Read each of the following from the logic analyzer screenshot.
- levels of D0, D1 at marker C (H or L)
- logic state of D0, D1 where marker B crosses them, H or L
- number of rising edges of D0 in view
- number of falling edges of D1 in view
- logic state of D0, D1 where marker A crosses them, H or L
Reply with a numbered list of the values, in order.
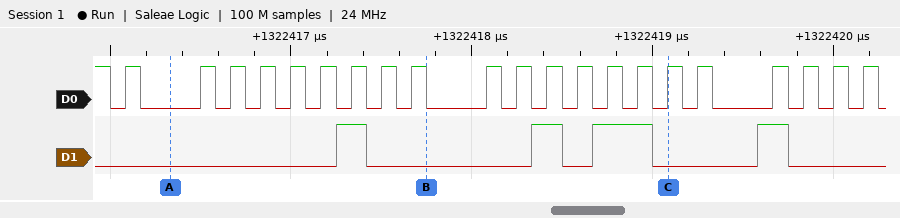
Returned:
1. D0=H, D1=L
2. D0=L, D1=L
3. 21
4. 4
5. D0=L, D1=L
